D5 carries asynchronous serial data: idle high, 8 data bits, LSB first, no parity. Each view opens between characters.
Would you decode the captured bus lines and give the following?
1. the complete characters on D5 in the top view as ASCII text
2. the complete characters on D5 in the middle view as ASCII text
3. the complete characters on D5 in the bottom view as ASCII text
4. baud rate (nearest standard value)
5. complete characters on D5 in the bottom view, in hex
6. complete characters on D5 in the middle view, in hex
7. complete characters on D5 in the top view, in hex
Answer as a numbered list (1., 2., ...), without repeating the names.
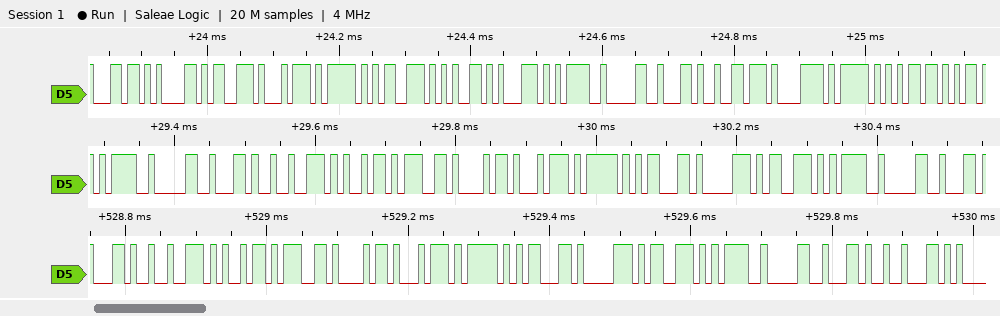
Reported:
1. "last_seq=0,vx_m"
2. "=0,right_cps=0"
3. ",right_cps=0,b"
4. 115200 baud
5. 2C, 72, 69, 67, 68, 74, 5F, 63, 70, 73, 3D, 30, 2C, 62
6. 3D, 30, 2C, 72, 69, 67, 68, 74, 5F, 63, 70, 73, 3D, 30
7. 6C, 61, 73, 74, 5F, 73, 65, 71, 3D, 30, 2C, 76, 78, 5F, 6D
